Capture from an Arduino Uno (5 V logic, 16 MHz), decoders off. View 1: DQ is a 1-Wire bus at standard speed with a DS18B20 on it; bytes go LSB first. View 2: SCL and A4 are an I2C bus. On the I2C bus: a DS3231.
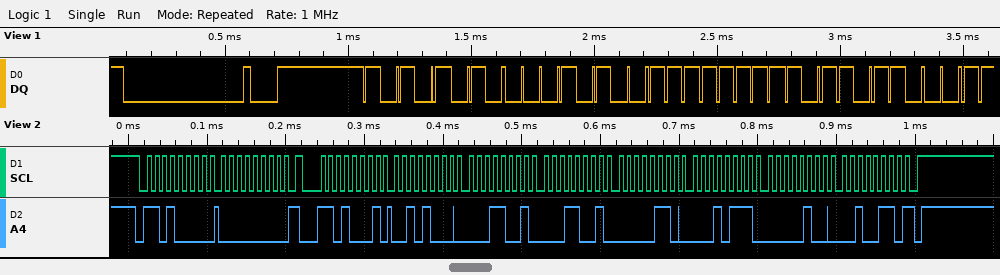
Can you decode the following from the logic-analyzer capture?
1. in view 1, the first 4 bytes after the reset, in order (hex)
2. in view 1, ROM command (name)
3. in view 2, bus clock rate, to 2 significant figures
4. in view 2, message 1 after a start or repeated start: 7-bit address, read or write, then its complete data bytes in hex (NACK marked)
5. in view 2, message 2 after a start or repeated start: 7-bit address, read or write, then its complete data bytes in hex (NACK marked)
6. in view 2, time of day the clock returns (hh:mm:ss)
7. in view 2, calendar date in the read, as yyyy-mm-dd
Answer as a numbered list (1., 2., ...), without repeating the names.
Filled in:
1. 55 28 FF 6D
2. Match ROM
3. 100 kHz
4. 0x68 write: 00
5. 0x68 read: 28 19 19 06 17 04 26 NACK
6. 19:19:28
7. 2026-04-17
